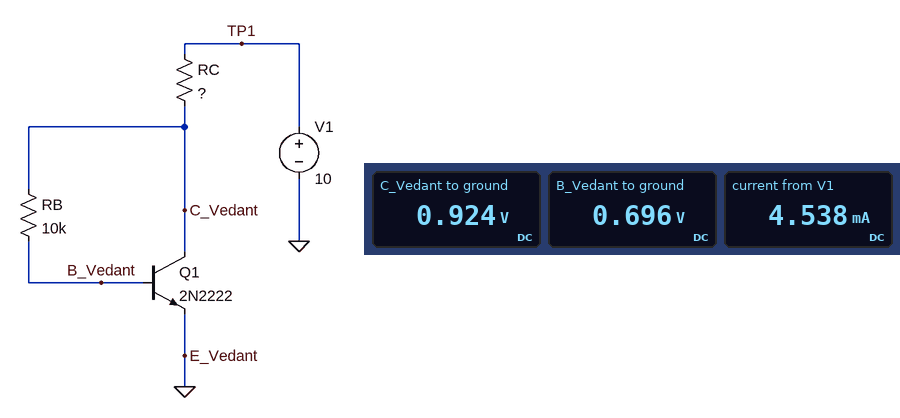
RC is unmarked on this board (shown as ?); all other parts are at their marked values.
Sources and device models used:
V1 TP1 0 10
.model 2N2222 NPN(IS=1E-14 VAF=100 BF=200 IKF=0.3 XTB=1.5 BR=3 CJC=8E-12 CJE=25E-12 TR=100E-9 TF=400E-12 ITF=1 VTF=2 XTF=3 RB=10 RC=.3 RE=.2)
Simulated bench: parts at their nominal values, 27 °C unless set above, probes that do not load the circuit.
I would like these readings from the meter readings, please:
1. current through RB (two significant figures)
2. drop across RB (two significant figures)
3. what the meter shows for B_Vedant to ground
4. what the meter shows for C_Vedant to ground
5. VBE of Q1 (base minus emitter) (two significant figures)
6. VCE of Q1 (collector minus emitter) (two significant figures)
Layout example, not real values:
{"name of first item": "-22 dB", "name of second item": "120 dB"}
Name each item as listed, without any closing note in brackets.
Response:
{"current through RB": "23 µA", "drop across RB": "230 mV", "what the meter shows for B_Vedant to ground": "0.696 V", "what the meter shows for C_Vedant to ground": "0.924 V", "VBE of Q1 (base minus emitter)": "700 mV", "VCE of Q1 (collector minus emitter)": "920 mV"}
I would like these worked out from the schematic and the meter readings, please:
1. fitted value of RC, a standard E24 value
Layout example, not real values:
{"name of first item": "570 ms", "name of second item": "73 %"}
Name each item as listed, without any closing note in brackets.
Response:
{"fitted value of RC, a standard E24 value": "2 kΩ"}
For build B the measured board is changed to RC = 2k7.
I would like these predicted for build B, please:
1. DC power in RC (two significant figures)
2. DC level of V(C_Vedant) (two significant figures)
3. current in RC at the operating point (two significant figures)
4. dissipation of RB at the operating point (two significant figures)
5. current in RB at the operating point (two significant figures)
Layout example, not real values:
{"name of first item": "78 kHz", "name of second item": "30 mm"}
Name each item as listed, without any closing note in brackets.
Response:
{"DC power in RC": "31 mW", "DC level of V(C_Vedant)": "860 mV", "current in RC at the operating point": "3.4 mA", "dissipation of RB at the operating point": "2.9 µW", "current in RB at the operating point": "17 µA"}
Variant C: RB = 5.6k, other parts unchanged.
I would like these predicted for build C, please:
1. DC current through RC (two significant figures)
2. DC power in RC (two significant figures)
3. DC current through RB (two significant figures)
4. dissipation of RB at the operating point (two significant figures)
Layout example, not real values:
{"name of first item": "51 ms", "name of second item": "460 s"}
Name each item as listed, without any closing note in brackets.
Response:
{"DC current through RC": "4.6 mA", "DC power in RC": "42 mW", "DC current through RB": "23 µA", "dissipation of RB at the operating point": "3.0 µW"}
